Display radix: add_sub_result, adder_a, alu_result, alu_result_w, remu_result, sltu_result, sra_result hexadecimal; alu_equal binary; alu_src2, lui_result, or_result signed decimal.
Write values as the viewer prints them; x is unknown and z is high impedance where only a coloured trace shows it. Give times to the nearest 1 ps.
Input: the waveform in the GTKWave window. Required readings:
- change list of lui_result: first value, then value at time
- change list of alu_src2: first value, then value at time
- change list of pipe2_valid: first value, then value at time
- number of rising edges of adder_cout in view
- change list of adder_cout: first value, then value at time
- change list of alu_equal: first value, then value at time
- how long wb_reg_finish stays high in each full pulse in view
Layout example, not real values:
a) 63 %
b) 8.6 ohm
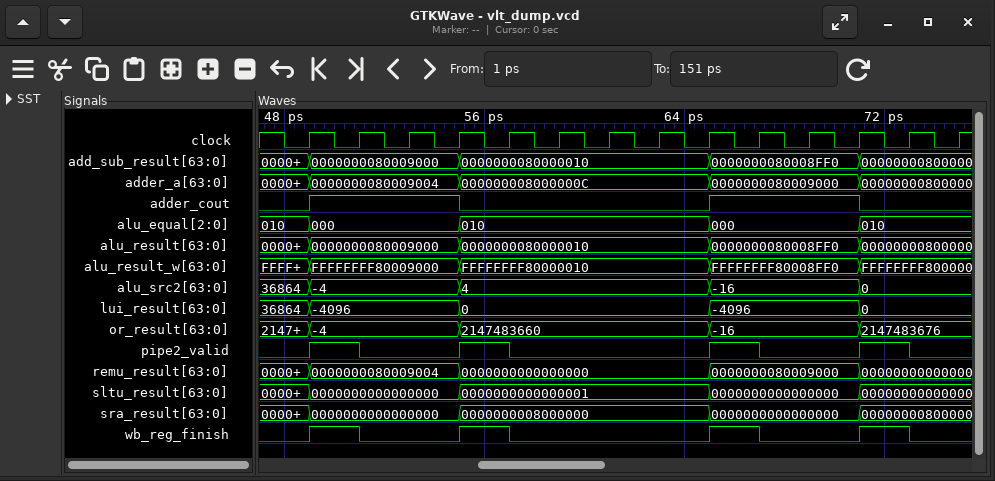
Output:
a) 36864, -4096 at 49 ps, 0 at 55 ps, -4096 at 65 ps, 0 at 71 ps
b) 36864, -4 at 49 ps, 4 at 55 ps, -16 at 65 ps, 0 at 71 ps
c) 0, 1 at 49 ps, 0 at 51 ps, 1 at 55 ps, 0 at 57 ps, 1 at 65 ps, 0 at 67 ps, 1 at 71 ps, 0 at 73 ps
d) 2
e) 0, 1 at 49 ps, 0 at 55 ps, 1 at 65 ps, 0 at 71 ps
f) 010, 000 at 49 ps, 010 at 55 ps, 000 at 65 ps, 010 at 71 ps
g) 2 ps, 2 ps, 2 ps, 2 ps
